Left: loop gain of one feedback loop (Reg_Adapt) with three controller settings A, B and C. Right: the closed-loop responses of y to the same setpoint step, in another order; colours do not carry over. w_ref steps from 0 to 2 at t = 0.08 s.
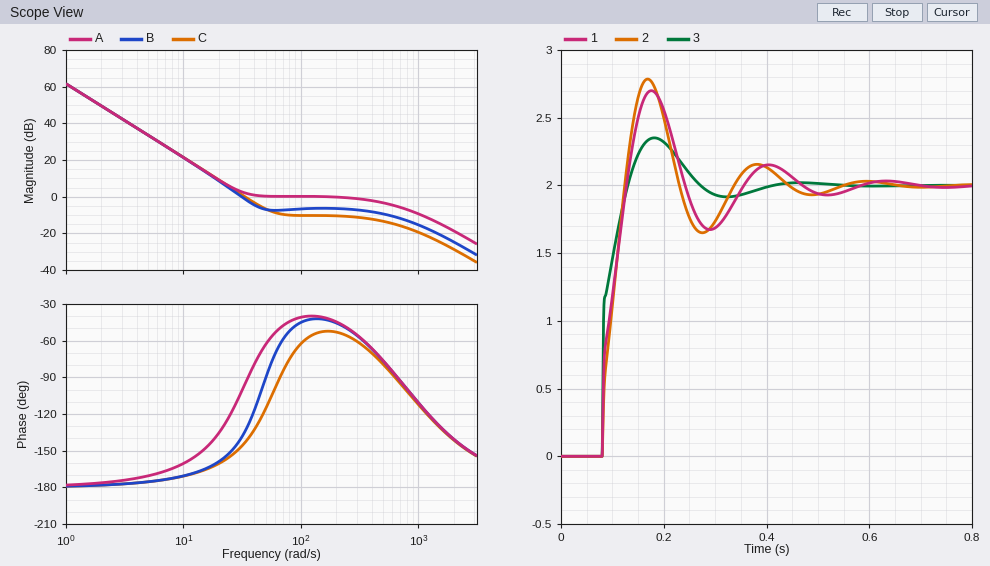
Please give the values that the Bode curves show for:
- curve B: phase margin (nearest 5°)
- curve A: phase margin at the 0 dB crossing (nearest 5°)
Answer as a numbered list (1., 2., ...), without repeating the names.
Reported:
1. 40°
2. 140°
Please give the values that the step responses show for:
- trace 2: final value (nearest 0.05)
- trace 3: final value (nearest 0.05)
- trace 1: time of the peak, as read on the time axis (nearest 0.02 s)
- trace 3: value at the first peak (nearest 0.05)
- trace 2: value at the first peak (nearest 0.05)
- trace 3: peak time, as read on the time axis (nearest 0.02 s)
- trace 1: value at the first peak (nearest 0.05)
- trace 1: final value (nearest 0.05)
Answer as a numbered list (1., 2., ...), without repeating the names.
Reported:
1. 2.00
2. 2.00
3. 0.18 s
4. 2.35
5. 2.80
6. 0.18 s
7. 2.70
8. 2.00
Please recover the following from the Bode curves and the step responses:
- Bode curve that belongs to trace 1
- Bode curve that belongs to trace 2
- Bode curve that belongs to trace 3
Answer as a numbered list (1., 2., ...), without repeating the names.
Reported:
1. B
2. C
3. A
